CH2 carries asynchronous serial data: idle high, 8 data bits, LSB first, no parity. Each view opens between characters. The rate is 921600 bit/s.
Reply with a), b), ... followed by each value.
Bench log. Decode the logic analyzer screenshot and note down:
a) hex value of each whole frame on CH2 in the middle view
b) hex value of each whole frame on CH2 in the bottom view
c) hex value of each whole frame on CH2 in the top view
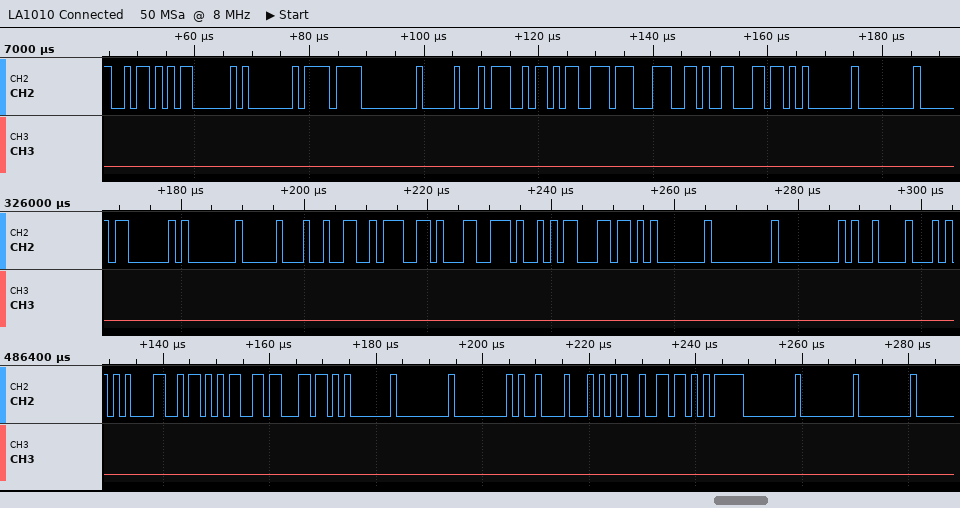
a) 03, 01, 10, 32, 67, CC, A9, 6C, 01, 00, 00, 09
b) 85, 5A, B3, 6C, 01, 00, 00, 09, 54, B2, F5, 00, 00, 00
c) 5A, 03, 01, EF, 00, 10, A7, CD, C7, 96, 6C, 01, 00
